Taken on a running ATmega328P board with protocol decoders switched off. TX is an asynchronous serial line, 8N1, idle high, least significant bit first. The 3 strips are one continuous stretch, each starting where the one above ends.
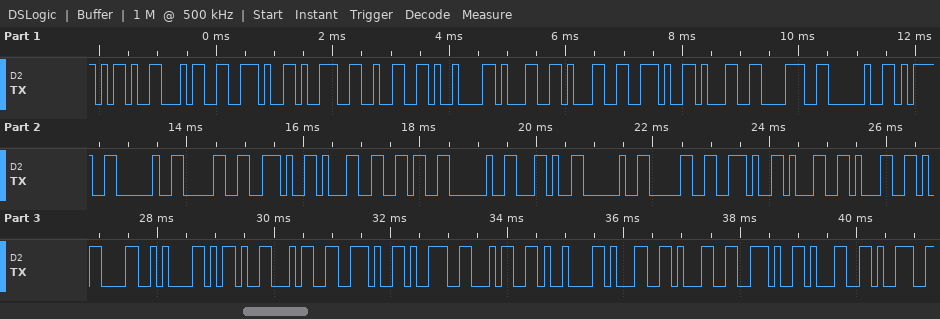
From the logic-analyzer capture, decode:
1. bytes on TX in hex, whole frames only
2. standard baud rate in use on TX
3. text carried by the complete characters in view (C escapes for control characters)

2D 34 2E 39 32 09 31 31 2E 31 38 20 3D 20 30 2E 31 36 20 2C 20 30 2E 31 31 0D 0A 2D 34 2E 39 34 09 31 31 2E 31 39
9600 baud
"-4.92\t11.18 = 0.16 , 0.11\r\n-4.94\t11.19"
